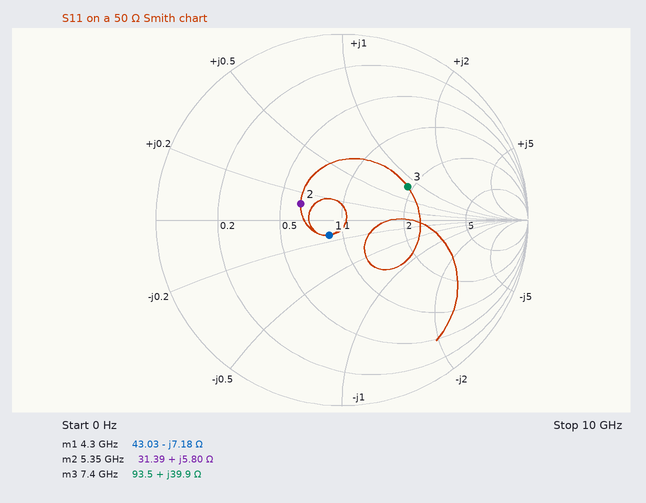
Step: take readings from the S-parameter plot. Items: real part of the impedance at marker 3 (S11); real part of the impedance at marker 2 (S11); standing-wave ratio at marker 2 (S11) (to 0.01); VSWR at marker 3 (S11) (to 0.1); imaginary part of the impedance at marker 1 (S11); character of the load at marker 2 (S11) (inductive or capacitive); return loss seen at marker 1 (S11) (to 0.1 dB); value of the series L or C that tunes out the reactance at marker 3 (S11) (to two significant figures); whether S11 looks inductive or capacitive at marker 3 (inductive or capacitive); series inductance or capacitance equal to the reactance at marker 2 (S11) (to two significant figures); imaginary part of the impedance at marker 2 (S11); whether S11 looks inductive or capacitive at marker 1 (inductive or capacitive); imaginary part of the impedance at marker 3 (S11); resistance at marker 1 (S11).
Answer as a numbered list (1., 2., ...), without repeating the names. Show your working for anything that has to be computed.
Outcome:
1. 93.5 Ω
2. 31.39 Ω
3. 1.63
4. 2.3
5. -7.18 Ω
6. inductive
7. 19.4 dB
8. C = 1/(2π × 7.4 GHz × 39.9 Ω) ≈ 539 fF, so 540 fF to two significant figures
9. inductive
10. L = 5.8 Ω/(2π × 5.35 GHz) ≈ 173 pH, so 170 pH to two significant figures
11. +5.80 Ω
12. capacitive
13. +39.9 Ω
14. 43.03 Ω
